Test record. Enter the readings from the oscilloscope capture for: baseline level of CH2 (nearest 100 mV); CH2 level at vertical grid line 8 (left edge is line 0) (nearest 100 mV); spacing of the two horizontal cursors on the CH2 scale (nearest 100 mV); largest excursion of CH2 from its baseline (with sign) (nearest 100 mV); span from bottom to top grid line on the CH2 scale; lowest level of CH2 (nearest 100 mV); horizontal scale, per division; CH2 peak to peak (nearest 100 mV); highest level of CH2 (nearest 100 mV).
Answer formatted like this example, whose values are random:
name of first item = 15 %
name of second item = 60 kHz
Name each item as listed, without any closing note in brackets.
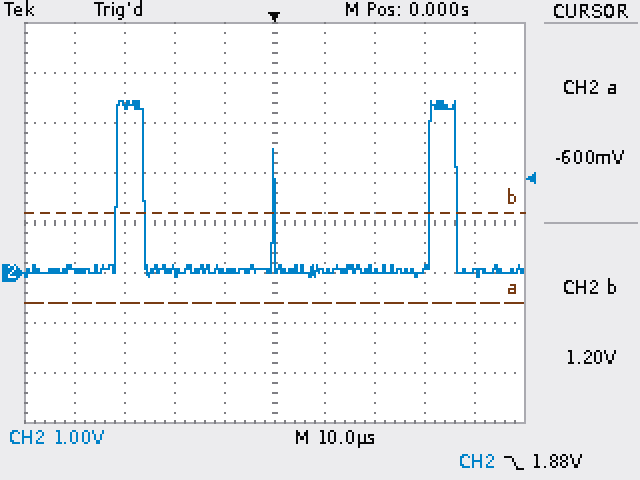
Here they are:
baseline level of CH2 = 0.0 V
CH2 level at vertical grid line 8 (left edge is line 0) = 100 mV
spacing of the two horizontal cursors on the CH2 scale = 1.8 V
largest excursion of CH2 from its baseline (with sign) = +3.4 V
span from bottom to top grid line on the CH2 scale = 8 V
lowest level of CH2 = -100 mV
horizontal scale, per division = 10 µs
CH2 peak to peak = 3.5 V
highest level of CH2 = 3.4 V
